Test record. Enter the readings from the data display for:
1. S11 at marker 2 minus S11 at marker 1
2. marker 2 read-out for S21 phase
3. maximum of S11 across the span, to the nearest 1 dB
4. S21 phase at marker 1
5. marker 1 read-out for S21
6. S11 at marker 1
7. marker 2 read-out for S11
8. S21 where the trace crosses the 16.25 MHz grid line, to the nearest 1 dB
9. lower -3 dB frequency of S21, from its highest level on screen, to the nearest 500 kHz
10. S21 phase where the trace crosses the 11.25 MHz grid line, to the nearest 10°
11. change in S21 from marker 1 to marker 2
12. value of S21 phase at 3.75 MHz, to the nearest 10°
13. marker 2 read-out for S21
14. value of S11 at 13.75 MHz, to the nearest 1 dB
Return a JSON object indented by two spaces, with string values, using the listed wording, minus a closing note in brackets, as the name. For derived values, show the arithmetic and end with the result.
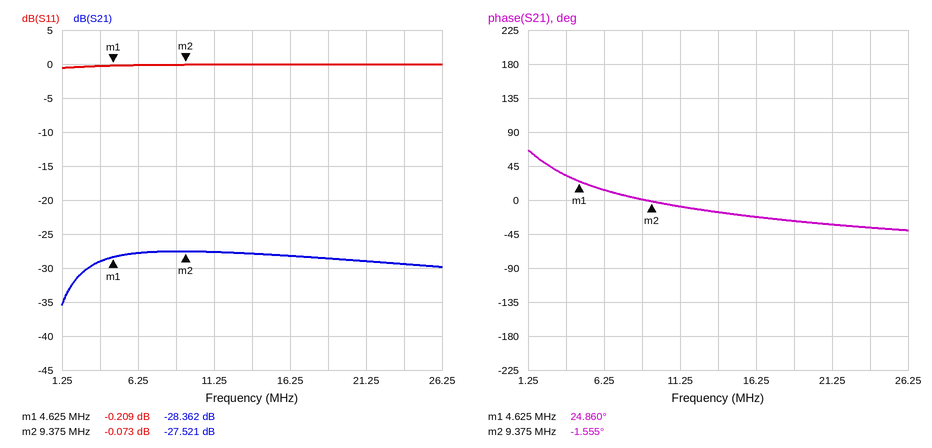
{
  "S11 at marker 2 minus S11 at marker 1": "-0.073 − (-0.209) = 0.136 dB",
  "marker 2 read-out for S21 phase": "-1.555°",
  "maximum of S11 across the span, to the nearest 1 dB": "0 dB",
  "S21 phase at marker 1": "24.860°",
  "marker 1 read-out for S21": "-28.362 dB",
  "S11 at marker 1": "-0.209 dB",
  "marker 2 read-out for S11": "-0.073 dB",
  "S21 where the trace crosses the 16.25 MHz grid line, to the nearest 1 dB": "-28 dB",
  "lower -3 dB frequency of S21, from its highest level on screen, to the nearest 500 kHz": "2.5 MHz",
  "S21 phase where the trace crosses the 11.25 MHz grid line, to the nearest 10°": "-10°",
  "change in S21 from marker 1 to marker 2": "-27.521 − (-28.362) = 0.841 dB",
  "value of S21 phase at 3.75 MHz, to the nearest 10°": "30°",
  "marker 2 read-out for S21": "-27.521 dB",
  "value of S11 at 13.75 MHz, to the nearest 1 dB": "0 dB"
}
